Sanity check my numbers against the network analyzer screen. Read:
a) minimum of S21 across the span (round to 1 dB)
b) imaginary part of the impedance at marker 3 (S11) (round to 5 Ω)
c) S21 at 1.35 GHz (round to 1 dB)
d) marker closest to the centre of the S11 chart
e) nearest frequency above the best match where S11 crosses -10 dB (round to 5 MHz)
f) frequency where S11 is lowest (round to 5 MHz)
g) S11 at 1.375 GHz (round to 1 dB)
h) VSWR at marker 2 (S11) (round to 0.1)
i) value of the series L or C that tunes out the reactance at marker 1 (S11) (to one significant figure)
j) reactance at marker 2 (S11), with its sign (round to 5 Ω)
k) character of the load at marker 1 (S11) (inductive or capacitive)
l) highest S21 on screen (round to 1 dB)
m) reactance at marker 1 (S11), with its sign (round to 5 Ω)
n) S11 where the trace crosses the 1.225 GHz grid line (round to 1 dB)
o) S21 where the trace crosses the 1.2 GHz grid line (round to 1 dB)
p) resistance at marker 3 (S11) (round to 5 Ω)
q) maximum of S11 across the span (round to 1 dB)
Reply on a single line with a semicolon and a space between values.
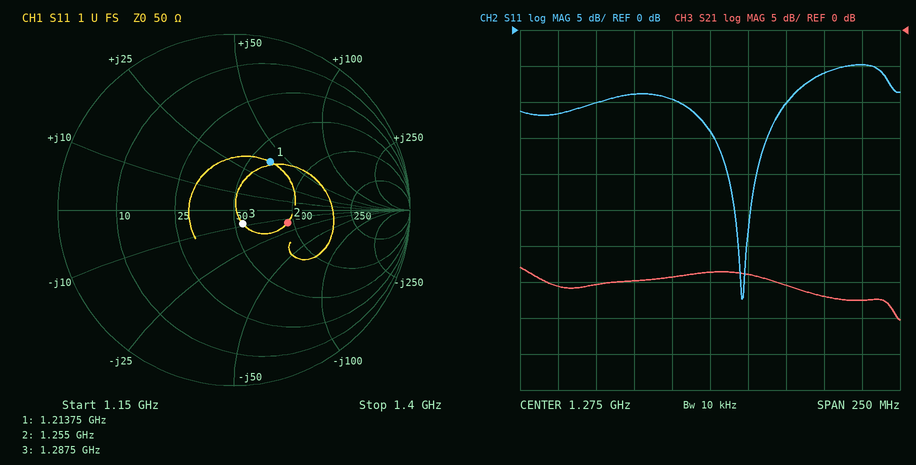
-40 dB; -10 Ω; -37 dB; marker 3; 1.325 GHz; 1.295 GHz; -5 dB; 1.9; 3 pF; -15 Ω; inductive; -33 dB; +40 Ω; -9 dB; -35 dB; 55 Ω; -5 dB
